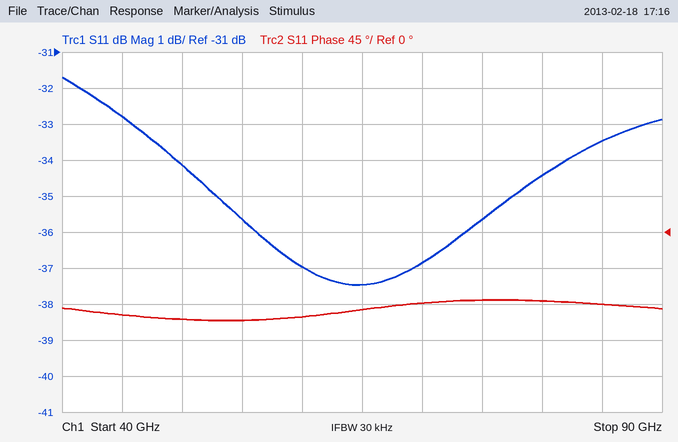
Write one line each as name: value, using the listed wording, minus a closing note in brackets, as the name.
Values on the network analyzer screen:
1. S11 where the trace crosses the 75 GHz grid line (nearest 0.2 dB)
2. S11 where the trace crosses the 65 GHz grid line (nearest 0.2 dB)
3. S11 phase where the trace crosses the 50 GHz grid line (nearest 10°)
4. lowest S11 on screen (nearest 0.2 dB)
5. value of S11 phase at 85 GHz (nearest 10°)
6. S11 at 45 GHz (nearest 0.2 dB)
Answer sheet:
S11 where the trace crosses the 75 GHz grid line: -35.6 dB
S11 where the trace crosses the 65 GHz grid line: -37.4 dB
S11 phase where the trace crosses the 50 GHz grid line: -110°
lowest S11 on screen: -37.4 dB
value of S11 phase at 85 GHz: -90°
S11 at 45 GHz: -32.8 dB
